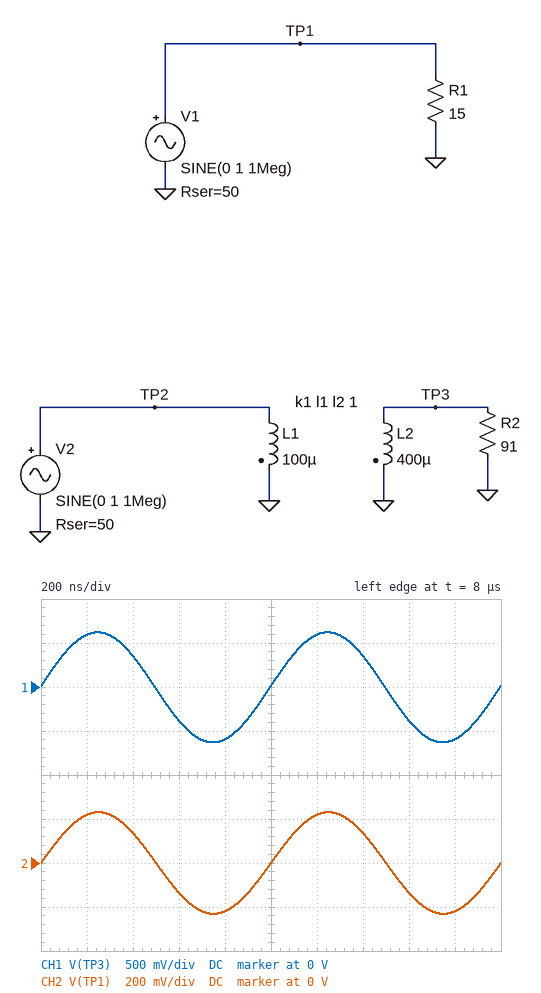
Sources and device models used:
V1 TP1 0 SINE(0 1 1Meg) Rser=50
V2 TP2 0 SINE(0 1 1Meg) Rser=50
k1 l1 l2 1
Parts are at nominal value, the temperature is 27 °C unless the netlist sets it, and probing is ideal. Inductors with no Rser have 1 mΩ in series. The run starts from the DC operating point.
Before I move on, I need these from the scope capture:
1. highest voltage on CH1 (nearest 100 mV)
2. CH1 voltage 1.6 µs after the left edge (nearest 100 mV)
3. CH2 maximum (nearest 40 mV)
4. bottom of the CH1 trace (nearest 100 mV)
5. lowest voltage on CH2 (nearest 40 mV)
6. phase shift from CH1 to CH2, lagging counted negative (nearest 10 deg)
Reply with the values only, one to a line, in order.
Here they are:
600 mV
-400 mV
240 mV
-600 mV
-240 mV
0 deg
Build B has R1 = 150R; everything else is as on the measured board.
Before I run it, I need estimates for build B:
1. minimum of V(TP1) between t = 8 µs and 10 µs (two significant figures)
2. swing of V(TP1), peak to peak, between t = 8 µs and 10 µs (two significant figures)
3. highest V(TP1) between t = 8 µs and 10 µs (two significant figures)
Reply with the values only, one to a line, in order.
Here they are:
-750 mV
1.5 V
750 mV
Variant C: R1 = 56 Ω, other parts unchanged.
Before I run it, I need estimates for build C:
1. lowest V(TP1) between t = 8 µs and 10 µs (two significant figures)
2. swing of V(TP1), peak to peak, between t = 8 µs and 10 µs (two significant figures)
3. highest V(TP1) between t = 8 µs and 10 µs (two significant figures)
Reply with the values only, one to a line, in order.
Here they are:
-530 mV
1.1 V
530 mV
